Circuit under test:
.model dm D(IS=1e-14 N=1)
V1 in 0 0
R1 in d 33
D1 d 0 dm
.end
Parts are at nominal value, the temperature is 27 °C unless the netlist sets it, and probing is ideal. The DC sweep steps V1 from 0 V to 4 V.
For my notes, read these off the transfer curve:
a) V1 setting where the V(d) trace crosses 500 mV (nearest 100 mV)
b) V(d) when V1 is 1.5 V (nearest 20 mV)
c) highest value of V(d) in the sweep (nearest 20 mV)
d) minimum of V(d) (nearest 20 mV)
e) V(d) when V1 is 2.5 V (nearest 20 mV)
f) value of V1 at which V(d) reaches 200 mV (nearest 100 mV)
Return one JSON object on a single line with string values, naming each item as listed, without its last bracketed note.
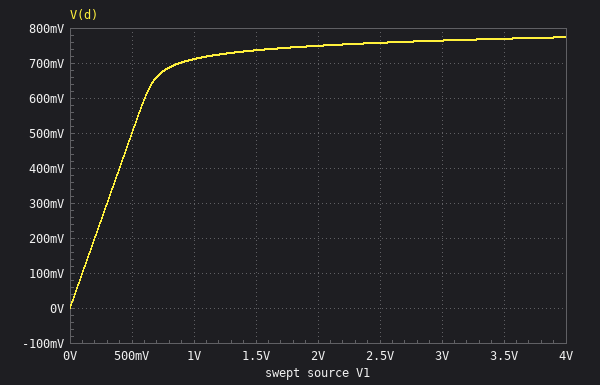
{"V1 setting where the V(d) trace crosses 500 mV": "500 mV", "V(d) when V1 is 1.5 V": "740 mV", "highest value of V(d) in the sweep": "780 mV", "minimum of V(d)": "0 V", "V(d) when V1 is 2.5 V": "760 mV", "value of V1 at which V(d) reaches 200 mV": "200 mV"}
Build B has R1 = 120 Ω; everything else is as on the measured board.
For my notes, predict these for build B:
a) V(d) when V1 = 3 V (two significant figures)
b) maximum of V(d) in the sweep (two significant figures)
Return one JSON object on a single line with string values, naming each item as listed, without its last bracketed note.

{"V(d) when V1 = 3 V": "730 mV", "maximum of V(d) in the sweep": "740 mV"}
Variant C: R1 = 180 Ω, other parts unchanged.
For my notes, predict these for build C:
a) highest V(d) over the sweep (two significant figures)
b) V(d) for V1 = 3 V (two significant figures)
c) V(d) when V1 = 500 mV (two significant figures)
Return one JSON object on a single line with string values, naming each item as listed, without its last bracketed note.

{"highest V(d) over the sweep": "730 mV", "V(d) for V1 = 3 V": "720 mV", "V(d) when V1 = 500 mV": "500 mV"}
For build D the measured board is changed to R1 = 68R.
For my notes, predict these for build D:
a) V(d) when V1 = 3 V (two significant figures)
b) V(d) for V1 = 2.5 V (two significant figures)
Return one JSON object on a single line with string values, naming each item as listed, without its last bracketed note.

{"V(d) when V1 = 3 V": "750 mV", "V(d) for V1 = 2.5 V": "740 mV"}
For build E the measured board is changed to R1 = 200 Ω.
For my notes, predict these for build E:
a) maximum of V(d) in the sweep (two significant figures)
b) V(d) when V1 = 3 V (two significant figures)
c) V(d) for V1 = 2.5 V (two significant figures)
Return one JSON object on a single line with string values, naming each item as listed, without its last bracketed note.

{"maximum of V(d) in the sweep": "730 mV", "V(d) when V1 = 3 V": "720 mV", "V(d) for V1 = 2.5 V": "710 mV"}
